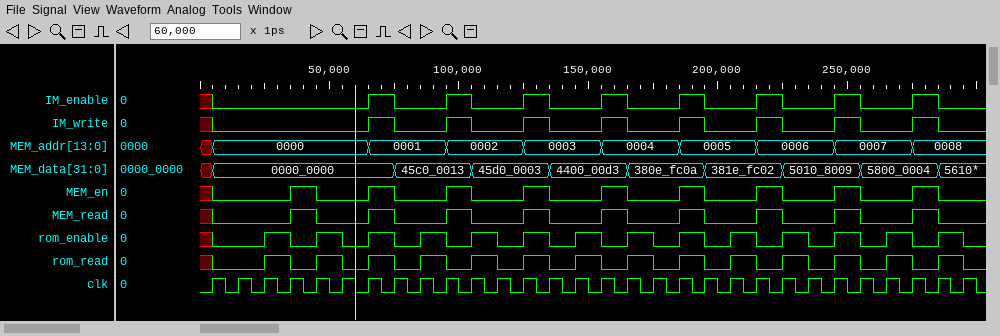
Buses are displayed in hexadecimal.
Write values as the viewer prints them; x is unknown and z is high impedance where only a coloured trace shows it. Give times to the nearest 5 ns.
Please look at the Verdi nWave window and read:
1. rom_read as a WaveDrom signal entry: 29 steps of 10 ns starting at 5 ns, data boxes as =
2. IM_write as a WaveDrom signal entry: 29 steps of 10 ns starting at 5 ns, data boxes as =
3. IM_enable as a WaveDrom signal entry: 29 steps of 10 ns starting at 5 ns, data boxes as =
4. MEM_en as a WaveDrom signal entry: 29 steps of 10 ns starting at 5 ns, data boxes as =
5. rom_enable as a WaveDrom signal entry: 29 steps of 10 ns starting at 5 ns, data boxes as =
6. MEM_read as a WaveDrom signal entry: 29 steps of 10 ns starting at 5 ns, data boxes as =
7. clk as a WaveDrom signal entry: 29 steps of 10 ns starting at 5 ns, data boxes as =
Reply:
{name: 'rom_read', wave: '0.101010101010101010101010101'}
{name: 'IM_write', wave: '0.....10.10.10.10.10.10.10.10'}
{name: 'IM_enable', wave: '0.....10.10.10.10.10.10.10.10'}
{name: 'MEM_en', wave: '0..10.10.10.10.10.10.10.10.10'}
{name: 'rom_enable', wave: '0.101010101010101010101010101'}
{name: 'MEM_read', wave: '0..10.10.10.10.10.10.10.10.10'}
{name: 'clk', wave: 'p............................'}
